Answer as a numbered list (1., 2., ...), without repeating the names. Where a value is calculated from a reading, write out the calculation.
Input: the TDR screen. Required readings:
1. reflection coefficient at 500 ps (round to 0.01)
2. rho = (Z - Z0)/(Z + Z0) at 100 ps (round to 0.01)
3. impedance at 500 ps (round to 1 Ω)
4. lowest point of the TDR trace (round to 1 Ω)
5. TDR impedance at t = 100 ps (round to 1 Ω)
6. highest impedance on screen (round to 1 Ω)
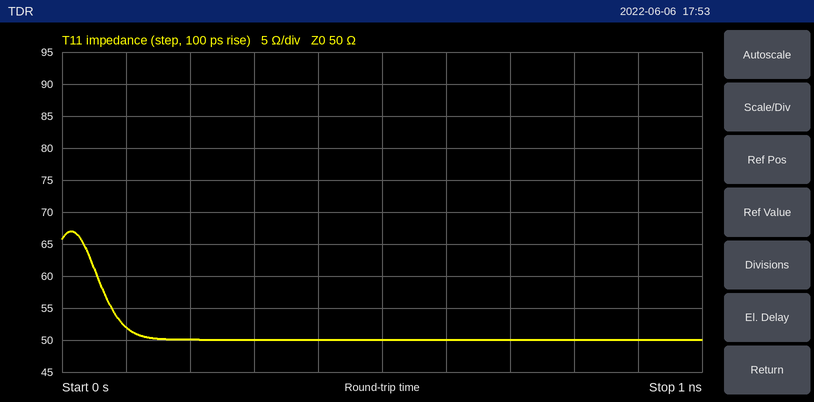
1. (50 − 50)/(50 + 50) ≈ 0.00
2. (52 − 50)/(52 + 50) ≈ +0.02
3. 50 Ω
4. 50 Ω
5. 52 Ω
6. 67 Ω
